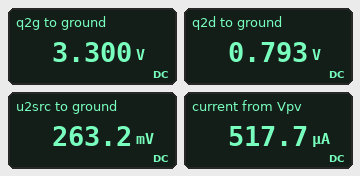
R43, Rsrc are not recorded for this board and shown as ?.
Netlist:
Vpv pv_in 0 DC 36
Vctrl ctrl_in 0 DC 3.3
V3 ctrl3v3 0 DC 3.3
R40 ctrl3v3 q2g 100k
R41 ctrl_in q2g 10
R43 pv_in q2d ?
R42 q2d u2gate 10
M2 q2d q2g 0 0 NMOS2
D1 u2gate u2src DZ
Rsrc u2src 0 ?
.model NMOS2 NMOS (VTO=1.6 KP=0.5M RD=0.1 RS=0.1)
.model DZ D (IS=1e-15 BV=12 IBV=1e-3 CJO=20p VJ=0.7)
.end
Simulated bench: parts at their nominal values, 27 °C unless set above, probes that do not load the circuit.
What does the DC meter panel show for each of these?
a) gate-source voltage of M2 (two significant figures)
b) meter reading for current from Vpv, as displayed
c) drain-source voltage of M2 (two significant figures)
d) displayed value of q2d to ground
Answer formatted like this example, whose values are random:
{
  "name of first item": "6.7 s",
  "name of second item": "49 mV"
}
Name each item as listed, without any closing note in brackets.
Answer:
{
  "gate-source voltage of M2": "3.3 V",
  "meter reading for current from Vpv, as displayed": "517.7 µA",
  "drain-source voltage of M2": "790 mV",
  "displayed value of q2d to ground": "0.793 V"
}
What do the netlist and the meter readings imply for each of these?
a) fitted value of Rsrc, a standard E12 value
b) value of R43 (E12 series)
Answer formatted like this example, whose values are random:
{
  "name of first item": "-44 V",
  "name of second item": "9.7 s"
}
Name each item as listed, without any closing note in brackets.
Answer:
{
  "fitted value of Rsrc, a standard E12 value": "330 kΩ",
  "value of R43": "68 kΩ"
}
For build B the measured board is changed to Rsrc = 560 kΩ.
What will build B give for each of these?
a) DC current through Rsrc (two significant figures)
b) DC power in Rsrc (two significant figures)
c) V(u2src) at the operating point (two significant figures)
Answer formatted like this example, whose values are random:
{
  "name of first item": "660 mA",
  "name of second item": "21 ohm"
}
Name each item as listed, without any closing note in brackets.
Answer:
{
  "DC current through Rsrc": "490 nA",
  "DC power in Rsrc": "140 nW",
  "V(u2src) at the operating point": "280 mV"
}
